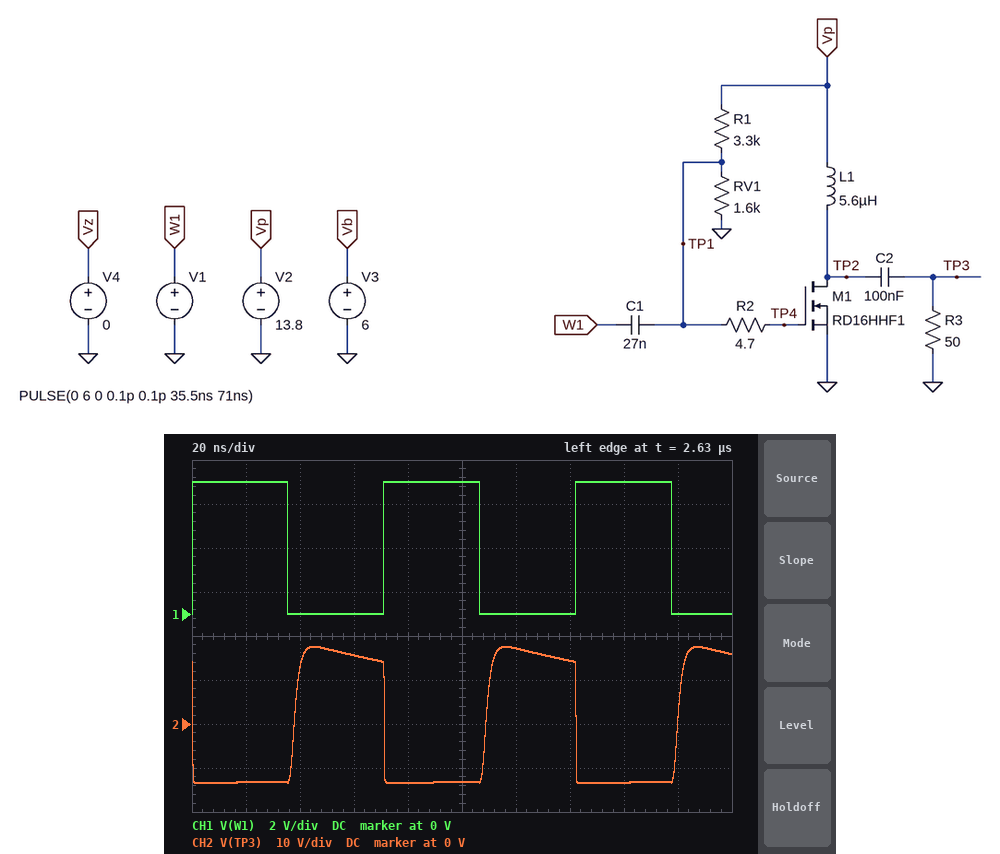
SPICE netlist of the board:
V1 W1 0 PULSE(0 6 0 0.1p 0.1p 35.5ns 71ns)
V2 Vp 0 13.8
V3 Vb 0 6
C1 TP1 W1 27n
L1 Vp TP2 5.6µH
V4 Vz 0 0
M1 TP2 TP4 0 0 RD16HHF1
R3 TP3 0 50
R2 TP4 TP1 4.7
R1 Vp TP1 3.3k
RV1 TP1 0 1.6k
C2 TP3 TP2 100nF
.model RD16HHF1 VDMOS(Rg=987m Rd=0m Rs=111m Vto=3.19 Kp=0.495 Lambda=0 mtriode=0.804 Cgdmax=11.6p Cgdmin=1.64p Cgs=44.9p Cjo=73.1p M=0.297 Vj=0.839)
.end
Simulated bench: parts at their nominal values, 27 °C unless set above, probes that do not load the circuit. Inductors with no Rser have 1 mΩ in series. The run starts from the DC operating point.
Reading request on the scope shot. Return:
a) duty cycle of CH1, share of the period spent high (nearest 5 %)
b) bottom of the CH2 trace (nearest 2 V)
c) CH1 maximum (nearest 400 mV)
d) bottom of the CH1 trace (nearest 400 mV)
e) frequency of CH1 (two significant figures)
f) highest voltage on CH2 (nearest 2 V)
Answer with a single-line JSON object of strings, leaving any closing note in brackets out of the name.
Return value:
{"duty cycle of CH1, share of the period spent high": "50 %", "bottom of the CH2 trace": "-14 V", "CH1 maximum": "6.0 V", "bottom of the CH1 trace": "0 V", "frequency of CH1": "14 MHz", "highest voltage on CH2": "18 V"}
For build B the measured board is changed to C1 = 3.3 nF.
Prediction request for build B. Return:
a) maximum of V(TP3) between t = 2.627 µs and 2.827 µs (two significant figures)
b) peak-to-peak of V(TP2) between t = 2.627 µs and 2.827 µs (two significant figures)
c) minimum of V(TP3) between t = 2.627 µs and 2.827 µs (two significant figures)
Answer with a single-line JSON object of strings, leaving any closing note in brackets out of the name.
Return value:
{"maximum of V(TP3) between t = 2.627 µs and 2.827 µs": "16 V", "peak-to-peak of V(TP2) between t = 2.627 µs and 2.827 µs": "30 V", "minimum of V(TP3) between t = 2.627 µs and 2.827 µs": "-14 V"}
